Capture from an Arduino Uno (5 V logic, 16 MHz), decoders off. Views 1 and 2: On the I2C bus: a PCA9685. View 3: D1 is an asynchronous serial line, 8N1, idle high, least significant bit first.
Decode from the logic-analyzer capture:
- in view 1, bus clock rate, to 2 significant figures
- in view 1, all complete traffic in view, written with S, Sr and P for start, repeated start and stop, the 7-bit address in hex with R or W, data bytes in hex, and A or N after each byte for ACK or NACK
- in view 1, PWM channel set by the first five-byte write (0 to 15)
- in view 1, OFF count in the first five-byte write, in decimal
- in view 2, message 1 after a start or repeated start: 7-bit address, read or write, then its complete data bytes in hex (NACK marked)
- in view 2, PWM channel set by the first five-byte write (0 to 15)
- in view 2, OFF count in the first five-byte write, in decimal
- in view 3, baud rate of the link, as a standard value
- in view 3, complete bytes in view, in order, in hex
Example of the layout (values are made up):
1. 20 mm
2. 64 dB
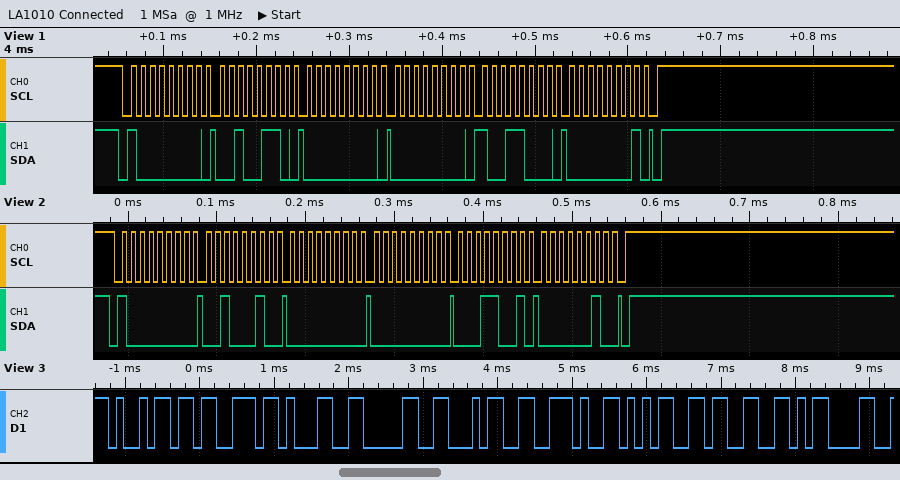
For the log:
1. 100 kHz
2. S 40W A 26 A 00 A 00 A 98 A 01 A P
3. 8
4. 408
5. 0x40 write: 22 00 00 19 02
6. 7
7. 537
8. 9600 baud
9. 69 73 31 30 34 2E 35 33 0D
